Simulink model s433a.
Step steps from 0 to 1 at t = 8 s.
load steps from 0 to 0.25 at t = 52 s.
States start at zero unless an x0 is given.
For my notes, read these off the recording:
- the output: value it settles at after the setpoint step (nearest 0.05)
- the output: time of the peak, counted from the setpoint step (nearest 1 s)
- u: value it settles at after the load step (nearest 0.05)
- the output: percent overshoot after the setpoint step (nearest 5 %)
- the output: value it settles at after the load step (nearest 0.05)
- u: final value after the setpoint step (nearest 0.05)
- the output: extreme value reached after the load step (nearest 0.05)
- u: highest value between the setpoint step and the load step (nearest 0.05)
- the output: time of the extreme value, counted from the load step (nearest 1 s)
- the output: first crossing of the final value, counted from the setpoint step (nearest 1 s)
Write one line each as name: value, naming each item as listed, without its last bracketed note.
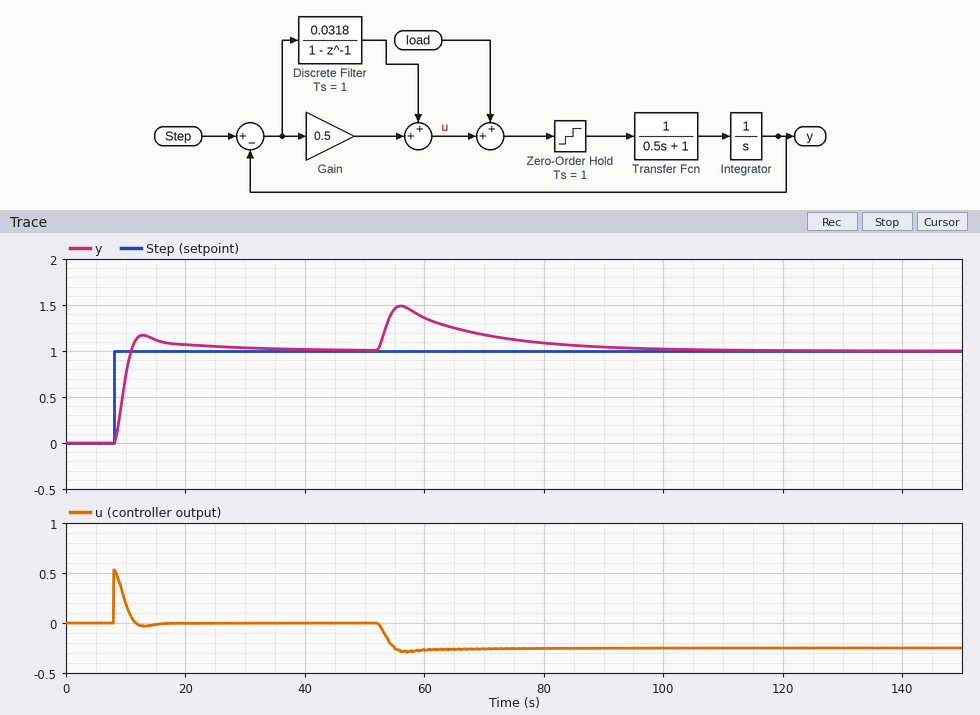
the output: value it settles at after the setpoint step: 1.00
the output: time of the peak, counted from the setpoint step: 5 s
u: value it settles at after the load step: -0.25
the output: percent overshoot after the setpoint step: 15 %
the output: value it settles at after the load step: 1.00
u: final value after the setpoint step: 0.00
the output: extreme value reached after the load step: 1.50
u: highest value between the setpoint step and the load step: 0.55
the output: time of the extreme value, counted from the load step: 4 s
the output: first crossing of the final value, counted from the setpoint step: 3 s
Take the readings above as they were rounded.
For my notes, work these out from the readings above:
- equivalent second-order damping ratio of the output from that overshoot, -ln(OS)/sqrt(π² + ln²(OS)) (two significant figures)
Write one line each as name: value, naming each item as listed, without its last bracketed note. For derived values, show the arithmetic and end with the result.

equivalent second-order damping ratio of the output from that overshoot, -ln(OS)/sqrt(π² + ln²(OS)): ln(0.15) = -1.897; 1.897 / sqrt(9.870 + 3.599) = 0.52
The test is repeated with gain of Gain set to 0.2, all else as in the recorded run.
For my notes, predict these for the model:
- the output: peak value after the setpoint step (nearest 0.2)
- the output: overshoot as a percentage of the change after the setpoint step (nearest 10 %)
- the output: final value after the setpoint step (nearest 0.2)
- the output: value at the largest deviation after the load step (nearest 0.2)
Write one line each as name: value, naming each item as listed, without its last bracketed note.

the output: peak value after the setpoint step: 1.4
the output: overshoot as a percentage of the change after the setpoint step: 30 %
the output: final value after the setpoint step: 1.0
the output: value at the largest deviation after the load step: 1.8
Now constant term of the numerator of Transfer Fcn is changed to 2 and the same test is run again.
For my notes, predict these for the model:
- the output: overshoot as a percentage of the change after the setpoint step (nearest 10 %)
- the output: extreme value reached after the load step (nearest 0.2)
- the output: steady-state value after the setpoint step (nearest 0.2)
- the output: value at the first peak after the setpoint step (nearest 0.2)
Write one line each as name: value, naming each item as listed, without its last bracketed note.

the output: overshoot as a percentage of the change after the setpoint step: 40 %
the output: extreme value reached after the load step: 1.6
the output: steady-state value after the setpoint step: 1.0
the output: value at the first peak after the setpoint step: 1.4
